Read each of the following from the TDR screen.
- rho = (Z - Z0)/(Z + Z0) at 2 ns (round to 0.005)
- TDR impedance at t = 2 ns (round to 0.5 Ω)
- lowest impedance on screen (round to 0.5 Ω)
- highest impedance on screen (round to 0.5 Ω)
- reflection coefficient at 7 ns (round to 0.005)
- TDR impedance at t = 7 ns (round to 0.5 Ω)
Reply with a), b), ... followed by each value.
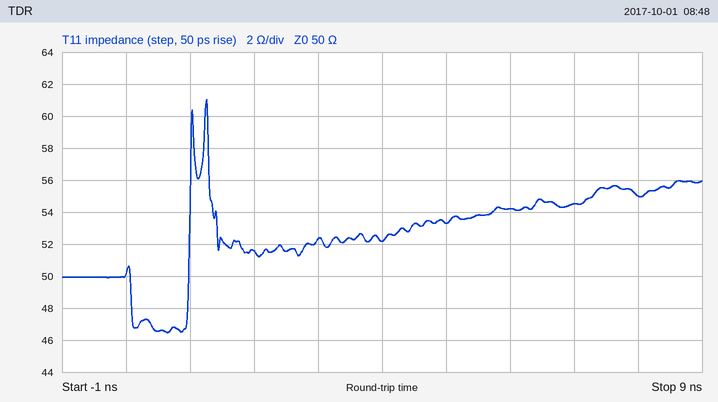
a) +0.015
b) 51.5 Ω
c) 46.5 Ω
d) 61.0 Ω
e) +0.045
f) 54.5 Ω
